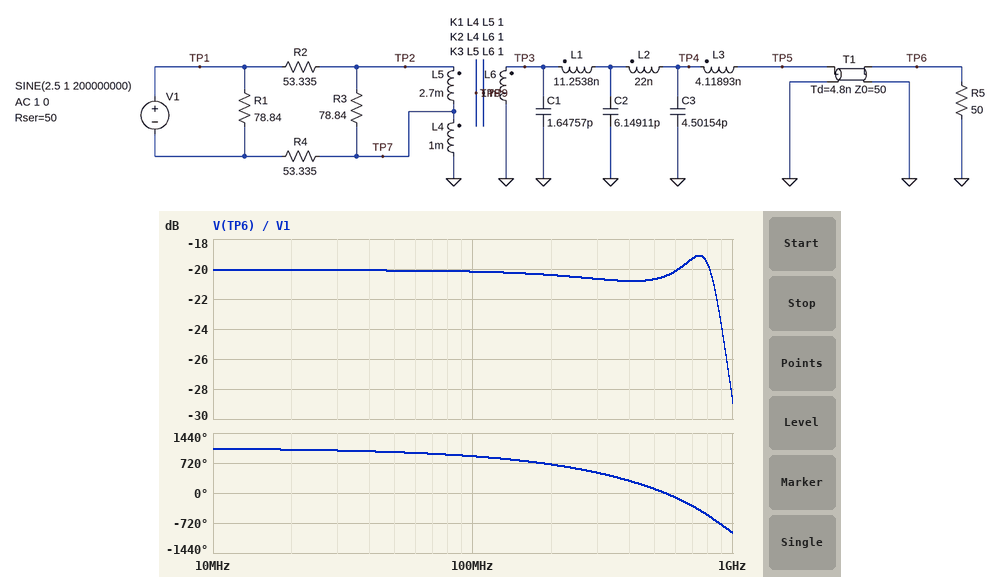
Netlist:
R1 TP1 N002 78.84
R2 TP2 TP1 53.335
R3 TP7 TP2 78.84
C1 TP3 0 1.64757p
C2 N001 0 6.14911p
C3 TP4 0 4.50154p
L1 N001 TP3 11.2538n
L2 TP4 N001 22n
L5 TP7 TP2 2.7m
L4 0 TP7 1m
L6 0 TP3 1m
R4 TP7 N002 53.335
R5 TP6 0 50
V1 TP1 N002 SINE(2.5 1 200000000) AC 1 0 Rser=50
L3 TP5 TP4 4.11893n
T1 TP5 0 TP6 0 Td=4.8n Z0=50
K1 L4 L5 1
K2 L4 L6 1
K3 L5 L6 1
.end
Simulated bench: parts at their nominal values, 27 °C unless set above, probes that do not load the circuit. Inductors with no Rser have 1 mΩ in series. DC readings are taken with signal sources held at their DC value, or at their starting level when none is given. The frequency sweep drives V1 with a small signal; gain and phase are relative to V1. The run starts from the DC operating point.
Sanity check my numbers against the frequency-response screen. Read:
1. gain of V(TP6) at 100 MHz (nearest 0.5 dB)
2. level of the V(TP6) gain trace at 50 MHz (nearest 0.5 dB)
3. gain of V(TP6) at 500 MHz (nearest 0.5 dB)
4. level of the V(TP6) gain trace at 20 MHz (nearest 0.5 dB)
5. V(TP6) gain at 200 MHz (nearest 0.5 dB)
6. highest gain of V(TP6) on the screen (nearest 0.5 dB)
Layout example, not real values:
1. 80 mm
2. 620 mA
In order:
1. -20.0 dB
2. -20.0 dB
3. -20.5 dB
4. -20.0 dB
5. -20.5 dB
6. -19.0 dB
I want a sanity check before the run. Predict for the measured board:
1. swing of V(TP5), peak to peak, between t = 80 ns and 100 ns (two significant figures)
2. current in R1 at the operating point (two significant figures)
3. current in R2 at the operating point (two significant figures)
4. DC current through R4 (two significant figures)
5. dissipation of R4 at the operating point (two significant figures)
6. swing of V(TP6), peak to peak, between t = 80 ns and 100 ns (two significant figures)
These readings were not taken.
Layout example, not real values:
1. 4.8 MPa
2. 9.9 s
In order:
1. 190 mV
2. 15 mA
3. 11 mA
4. 11 mA
5. 6.6 mW
6. 190 mV
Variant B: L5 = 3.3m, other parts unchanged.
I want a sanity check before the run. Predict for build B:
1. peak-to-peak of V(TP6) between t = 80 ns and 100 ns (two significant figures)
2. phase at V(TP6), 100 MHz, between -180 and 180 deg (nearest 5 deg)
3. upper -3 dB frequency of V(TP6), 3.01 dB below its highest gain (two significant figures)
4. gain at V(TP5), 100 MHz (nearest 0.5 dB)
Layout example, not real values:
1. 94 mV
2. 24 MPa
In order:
1. 180 mV
2. 160 deg
3. 860 MHz
4. -20.5 dB
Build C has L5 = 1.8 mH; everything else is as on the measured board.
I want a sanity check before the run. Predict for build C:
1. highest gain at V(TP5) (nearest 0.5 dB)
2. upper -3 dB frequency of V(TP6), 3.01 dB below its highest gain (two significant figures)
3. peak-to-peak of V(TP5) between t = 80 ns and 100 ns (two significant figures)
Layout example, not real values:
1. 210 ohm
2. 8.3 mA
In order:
1. -19.5 dB
2. 880 MHz
3. 210 mV
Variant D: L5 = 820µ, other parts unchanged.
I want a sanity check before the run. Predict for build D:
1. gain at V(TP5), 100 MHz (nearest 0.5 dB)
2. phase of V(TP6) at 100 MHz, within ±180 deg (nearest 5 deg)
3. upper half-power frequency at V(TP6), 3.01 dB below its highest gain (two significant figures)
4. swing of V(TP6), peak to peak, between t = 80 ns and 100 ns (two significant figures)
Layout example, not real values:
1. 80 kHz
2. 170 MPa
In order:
1. -19.0 dB
2. 165 deg
3. 810 MHz
4. 220 mV
